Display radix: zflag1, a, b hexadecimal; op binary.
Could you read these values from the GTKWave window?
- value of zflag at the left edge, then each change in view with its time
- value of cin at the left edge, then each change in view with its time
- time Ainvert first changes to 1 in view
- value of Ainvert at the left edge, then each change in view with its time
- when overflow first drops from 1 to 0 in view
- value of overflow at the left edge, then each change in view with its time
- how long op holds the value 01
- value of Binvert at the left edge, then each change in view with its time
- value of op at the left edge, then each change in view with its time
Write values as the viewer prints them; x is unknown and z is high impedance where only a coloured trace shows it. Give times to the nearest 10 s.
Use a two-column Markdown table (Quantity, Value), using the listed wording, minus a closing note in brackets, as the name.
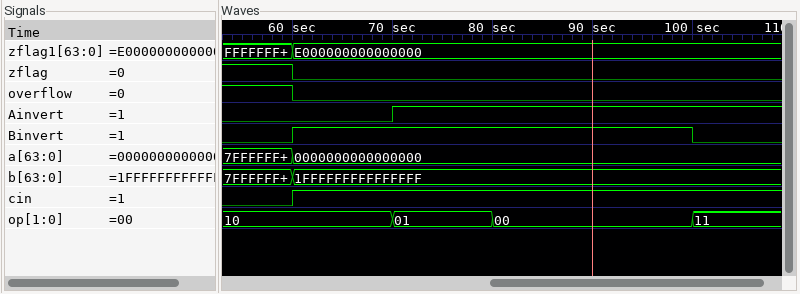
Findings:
| Quantity | Value |
|---|---|
| value of zflag at the left edge, then each change in view with its time | 1, 0 at 60 s |
| value of cin at the left edge, then each change in view with its time | 0, 1 at 60 s |
| time Ainvert first changes to 1 in view | 70 s |
| value of Ainvert at the left edge, then each change in view with its time | 0, 1 at 70 s |
| when overflow first drops from 1 to 0 in view | 60 s |
| value of overflow at the left edge, then each change in view with its time | 1, 0 at 60 s |
| how long op holds the value 01 | 10 s |
| value of Binvert at the left edge, then each change in view with its time | 0, 1 at 60 s, 0 at 100 s |
| value of op at the left edge, then each change in view with its time | 10, 01 at 70 s, 00 at 80 s, 11 at 100 s |
